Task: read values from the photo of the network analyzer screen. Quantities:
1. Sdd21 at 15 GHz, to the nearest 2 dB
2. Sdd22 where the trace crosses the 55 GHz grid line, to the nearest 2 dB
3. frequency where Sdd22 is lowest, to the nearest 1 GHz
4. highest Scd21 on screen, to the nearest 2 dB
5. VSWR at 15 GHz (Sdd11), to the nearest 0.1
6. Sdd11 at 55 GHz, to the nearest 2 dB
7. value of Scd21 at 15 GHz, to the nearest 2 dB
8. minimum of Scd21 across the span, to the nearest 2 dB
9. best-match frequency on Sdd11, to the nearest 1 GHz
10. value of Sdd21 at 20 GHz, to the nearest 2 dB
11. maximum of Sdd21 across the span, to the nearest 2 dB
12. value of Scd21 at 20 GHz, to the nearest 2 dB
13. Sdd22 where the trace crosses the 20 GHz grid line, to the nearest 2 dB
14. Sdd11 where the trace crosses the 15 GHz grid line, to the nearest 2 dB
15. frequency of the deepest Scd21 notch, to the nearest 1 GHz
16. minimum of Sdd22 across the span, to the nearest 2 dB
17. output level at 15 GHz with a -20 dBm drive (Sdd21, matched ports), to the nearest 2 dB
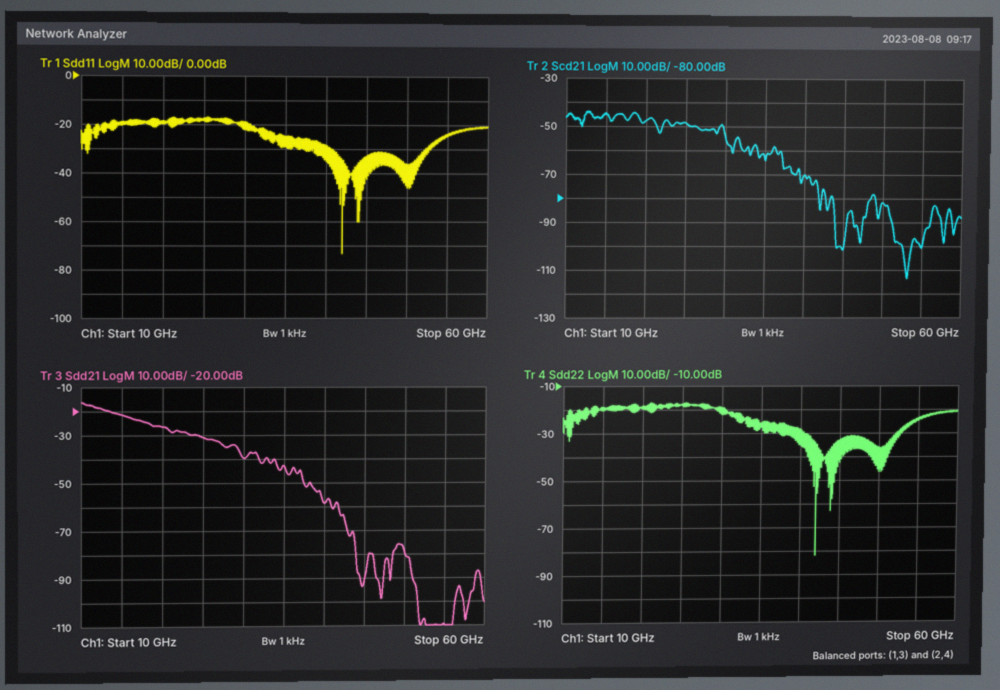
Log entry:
-22 dB
-24 dB
42 GHz
-44 dB
1.2
-24 dB
-44 dB
-114 dB
42 GHz
-26 dB
-16 dB
-48 dB
-20 dB
-20 dB
53 GHz
-82 dB
-42 dBm
